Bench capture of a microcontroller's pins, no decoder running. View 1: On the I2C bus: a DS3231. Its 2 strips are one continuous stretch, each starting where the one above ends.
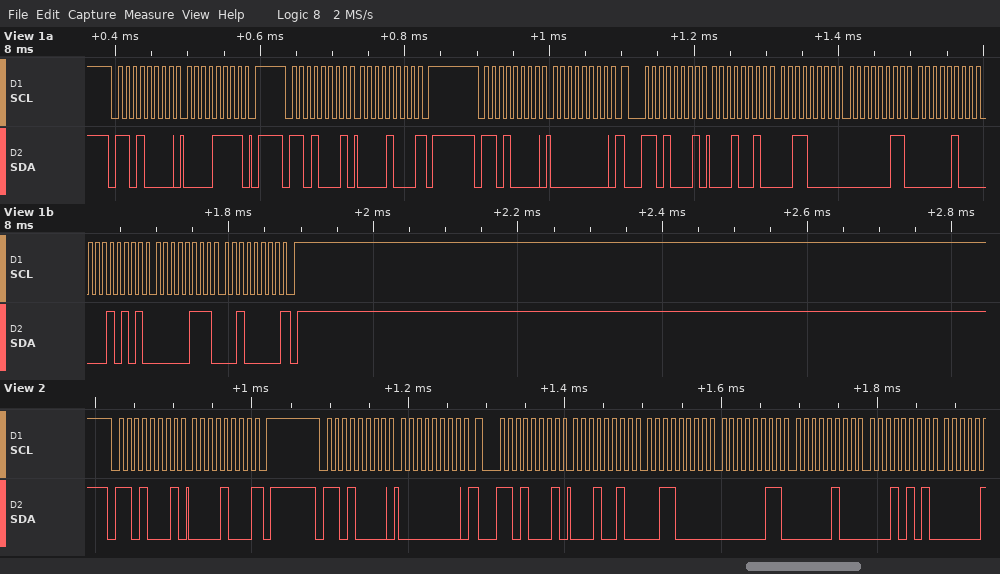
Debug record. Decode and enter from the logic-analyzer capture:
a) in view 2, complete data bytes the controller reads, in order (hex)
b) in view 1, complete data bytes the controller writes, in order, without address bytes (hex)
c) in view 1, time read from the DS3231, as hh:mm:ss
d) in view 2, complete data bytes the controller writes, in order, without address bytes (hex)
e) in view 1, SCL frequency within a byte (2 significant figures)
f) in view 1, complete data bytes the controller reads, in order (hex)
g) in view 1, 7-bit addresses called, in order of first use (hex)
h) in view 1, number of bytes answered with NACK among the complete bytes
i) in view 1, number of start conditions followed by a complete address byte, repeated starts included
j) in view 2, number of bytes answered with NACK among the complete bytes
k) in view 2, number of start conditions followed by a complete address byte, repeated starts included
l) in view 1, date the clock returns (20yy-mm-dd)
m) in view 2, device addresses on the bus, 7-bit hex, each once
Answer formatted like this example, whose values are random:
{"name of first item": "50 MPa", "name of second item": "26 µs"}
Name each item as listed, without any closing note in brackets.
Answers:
{"in view 2, complete data bytes the controller reads, in order": "08 12 30 03 04 15", "in view 1, complete data bytes the controller writes, in order, without address bytes": "0F 00", "in view 1, time read from the DS3231, as hh:mm:ss": "03:30:12", "in view 2, complete data bytes the controller writes, in order, without address bytes": "00", "in view 1, SCL frequency within a byte": "100 kHz", "in view 1, complete data bytes the controller reads, in order": "08 12 30 03 04 15 07 20", "in view 1, 7-bit addresses called, in order of first use": "0x68", "in view 1, number of bytes answered with NACK among the complete bytes": "2", "in view 1, number of start conditions followed by a complete address byte, repeated starts included": "4", "in view 2, number of bytes answered with NACK among the complete bytes": "1", "in view 2, number of start conditions followed by a complete address byte, repeated starts included": "3", "in view 1, date the clock returns": "2020-07-15", "in view 2, device addresses on the bus, 7-bit hex, each once": "0x68"}
